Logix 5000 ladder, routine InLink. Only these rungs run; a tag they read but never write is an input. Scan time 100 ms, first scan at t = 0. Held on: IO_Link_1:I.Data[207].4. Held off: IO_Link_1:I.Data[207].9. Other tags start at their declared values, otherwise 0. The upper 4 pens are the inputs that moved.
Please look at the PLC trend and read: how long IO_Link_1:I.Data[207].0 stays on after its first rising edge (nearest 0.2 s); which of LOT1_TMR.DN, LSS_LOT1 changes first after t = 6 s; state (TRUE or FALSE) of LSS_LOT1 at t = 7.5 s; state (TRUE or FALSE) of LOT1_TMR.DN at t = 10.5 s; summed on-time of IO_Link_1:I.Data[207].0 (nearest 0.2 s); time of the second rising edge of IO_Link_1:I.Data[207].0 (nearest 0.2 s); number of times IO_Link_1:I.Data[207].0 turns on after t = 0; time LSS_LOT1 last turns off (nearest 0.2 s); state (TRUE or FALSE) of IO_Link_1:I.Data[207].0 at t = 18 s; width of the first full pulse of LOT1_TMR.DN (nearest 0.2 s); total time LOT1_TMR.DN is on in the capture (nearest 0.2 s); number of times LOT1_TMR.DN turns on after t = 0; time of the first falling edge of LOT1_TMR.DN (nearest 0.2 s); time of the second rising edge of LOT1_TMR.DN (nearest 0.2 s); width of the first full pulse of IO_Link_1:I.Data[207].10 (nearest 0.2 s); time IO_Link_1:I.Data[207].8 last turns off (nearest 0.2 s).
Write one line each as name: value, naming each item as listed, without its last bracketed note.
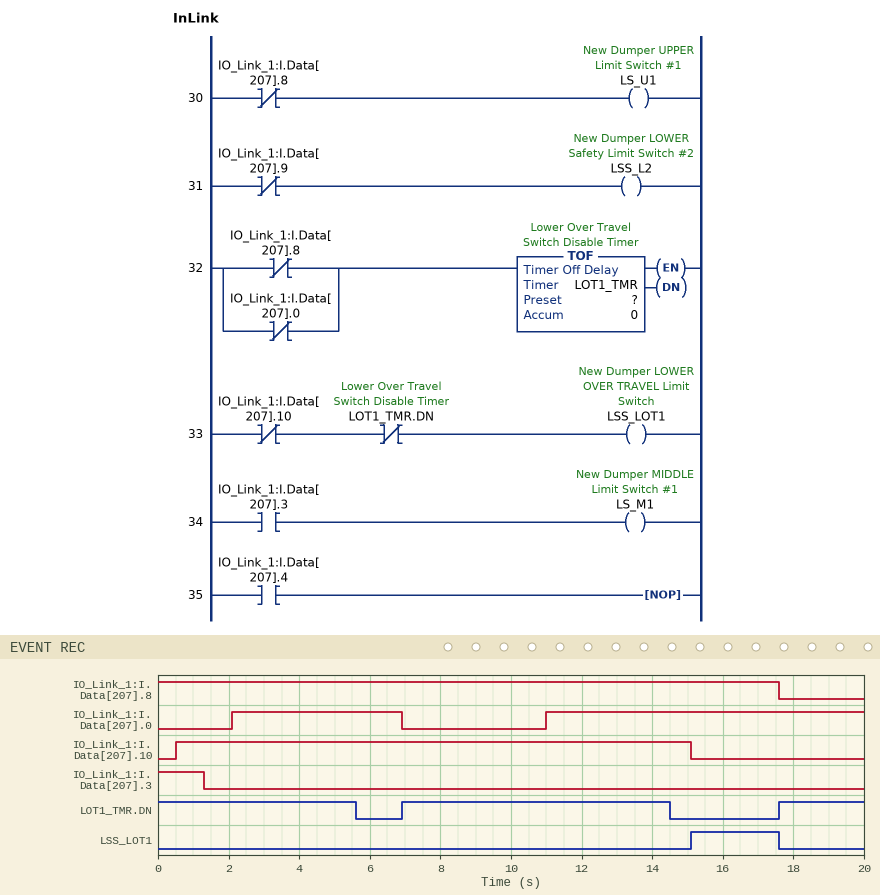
how long IO_Link_1:I.Data[207].0 stays on after its first rising edge: 4.8 s
which of LOT1_TMR.DN, LSS_LOT1 changes first after t = 6 s: LOT1_TMR.DN
state (TRUE or FALSE) of LSS_LOT1 at t = 7.5 s: FALSE
state (TRUE or FALSE) of LOT1_TMR.DN at t = 10.5 s: TRUE
summed on-time of IO_Link_1:I.Data[207].0: 13.8 s
time of the second rising edge of IO_Link_1:I.Data[207].0: 11.0 s
number of times IO_Link_1:I.Data[207].0 turns on after t = 0: 2
time LSS_LOT1 last turns off: 17.6 s
state (TRUE or FALSE) of IO_Link_1:I.Data[207].0 at t = 18 s: TRUE
width of the first full pulse of LOT1_TMR.DN: 7.6 s
total time LOT1_TMR.DN is on in the capture: 15.6 s
number of times LOT1_TMR.DN turns on after t = 0: 2
time of the first falling edge of LOT1_TMR.DN: 5.6 s
time of the second rising edge of LOT1_TMR.DN: 17.6 s
width of the first full pulse of IO_Link_1:I.Data[207].10: 14.6 s
time IO_Link_1:I.Data[207].8 last turns off: 17.6 s
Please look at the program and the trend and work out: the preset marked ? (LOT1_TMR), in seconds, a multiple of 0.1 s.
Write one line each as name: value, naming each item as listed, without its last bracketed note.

the preset marked ? (LOT1_TMR), in seconds, a multiple of 0.1 s: 3.5 s
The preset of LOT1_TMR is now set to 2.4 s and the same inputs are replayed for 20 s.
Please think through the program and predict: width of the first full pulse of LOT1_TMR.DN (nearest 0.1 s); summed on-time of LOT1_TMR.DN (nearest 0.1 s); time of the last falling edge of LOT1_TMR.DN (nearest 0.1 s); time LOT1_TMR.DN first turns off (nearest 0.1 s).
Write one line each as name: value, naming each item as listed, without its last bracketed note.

width of the first full pulse of LOT1_TMR.DN: 6.5 s
summed on-time of LOT1_TMR.DN: 13.4 s
time of the last falling edge of LOT1_TMR.DN: 13.4 s
time LOT1_TMR.DN first turns off: 4.5 s
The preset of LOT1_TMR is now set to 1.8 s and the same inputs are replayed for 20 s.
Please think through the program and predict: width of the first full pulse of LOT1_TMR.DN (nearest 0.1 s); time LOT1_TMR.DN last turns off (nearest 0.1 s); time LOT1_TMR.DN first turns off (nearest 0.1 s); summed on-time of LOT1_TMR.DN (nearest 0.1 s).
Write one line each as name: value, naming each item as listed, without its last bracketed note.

width of the first full pulse of LOT1_TMR.DN: 5.9 s
time LOT1_TMR.DN last turns off: 12.8 s
time LOT1_TMR.DN first turns off: 3.9 s
summed on-time of LOT1_TMR.DN: 12.2 s
